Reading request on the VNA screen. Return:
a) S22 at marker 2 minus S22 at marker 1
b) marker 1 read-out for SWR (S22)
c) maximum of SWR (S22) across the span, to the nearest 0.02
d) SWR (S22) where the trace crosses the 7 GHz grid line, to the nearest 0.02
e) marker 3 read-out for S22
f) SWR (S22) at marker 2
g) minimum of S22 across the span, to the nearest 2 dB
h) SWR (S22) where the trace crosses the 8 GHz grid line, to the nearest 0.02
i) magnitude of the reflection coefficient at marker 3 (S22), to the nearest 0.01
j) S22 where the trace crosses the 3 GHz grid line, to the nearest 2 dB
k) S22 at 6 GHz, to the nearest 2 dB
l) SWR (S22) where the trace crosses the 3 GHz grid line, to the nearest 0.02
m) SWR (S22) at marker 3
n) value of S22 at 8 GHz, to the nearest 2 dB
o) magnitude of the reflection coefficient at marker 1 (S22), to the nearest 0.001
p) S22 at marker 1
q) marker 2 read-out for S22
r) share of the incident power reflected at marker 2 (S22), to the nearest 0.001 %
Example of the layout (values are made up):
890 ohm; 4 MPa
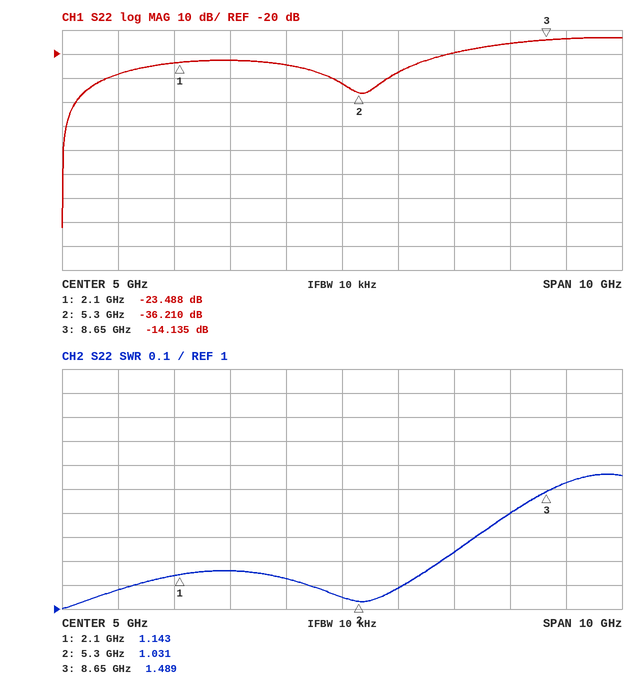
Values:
-12.722 dB; 1.143; 1.56; 1.24; -14.135 dB; 1.031; -92 dB; 1.40; 0.20; -22 dB; -28 dB; 1.16; 1.489; -16 dB; 0.067; -23.488 dB; -36.210 dB; 0.024 %
